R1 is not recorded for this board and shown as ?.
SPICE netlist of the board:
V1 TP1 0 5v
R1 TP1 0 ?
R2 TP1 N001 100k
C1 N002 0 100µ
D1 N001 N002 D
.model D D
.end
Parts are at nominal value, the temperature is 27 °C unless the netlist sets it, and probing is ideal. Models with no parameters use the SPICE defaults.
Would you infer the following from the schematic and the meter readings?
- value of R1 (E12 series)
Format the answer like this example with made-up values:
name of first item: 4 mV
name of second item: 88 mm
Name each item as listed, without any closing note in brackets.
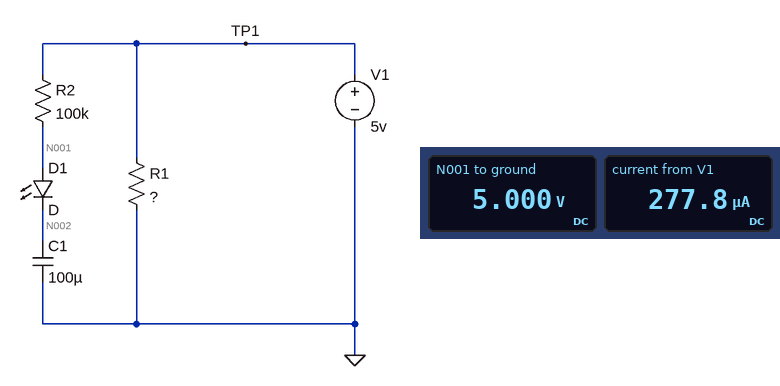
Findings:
value of R1: 18 kΩ
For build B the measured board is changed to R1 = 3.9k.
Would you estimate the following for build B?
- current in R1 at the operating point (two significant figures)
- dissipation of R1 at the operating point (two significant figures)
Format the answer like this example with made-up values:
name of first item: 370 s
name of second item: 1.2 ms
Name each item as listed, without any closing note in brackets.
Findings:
current in R1 at the operating point: 1.3 mA
dissipation of R1 at the operating point: 6.4 mW
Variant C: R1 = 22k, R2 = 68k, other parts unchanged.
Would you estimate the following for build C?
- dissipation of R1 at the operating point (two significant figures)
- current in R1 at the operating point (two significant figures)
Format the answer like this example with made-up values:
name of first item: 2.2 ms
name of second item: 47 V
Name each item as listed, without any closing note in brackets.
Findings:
dissipation of R1 at the operating point: 1.1 mW
current in R1 at the operating point: 230 µA
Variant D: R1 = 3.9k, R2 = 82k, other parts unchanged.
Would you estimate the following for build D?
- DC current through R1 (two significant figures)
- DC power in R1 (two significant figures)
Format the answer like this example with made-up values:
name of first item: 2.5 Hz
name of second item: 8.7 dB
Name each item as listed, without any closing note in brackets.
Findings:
DC current through R1: 1.3 mA
DC power in R1: 6.4 mW
